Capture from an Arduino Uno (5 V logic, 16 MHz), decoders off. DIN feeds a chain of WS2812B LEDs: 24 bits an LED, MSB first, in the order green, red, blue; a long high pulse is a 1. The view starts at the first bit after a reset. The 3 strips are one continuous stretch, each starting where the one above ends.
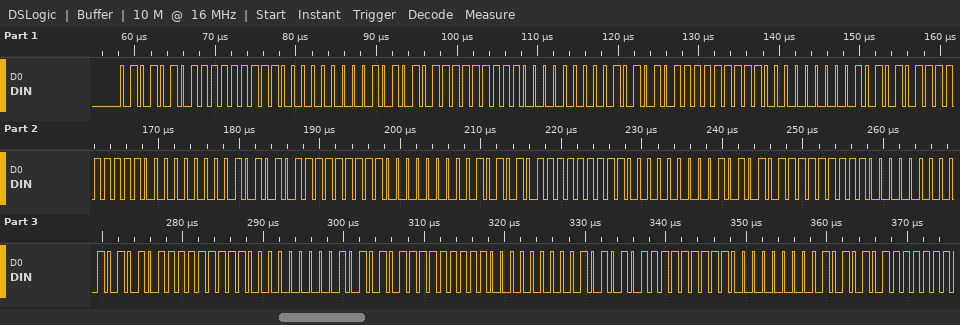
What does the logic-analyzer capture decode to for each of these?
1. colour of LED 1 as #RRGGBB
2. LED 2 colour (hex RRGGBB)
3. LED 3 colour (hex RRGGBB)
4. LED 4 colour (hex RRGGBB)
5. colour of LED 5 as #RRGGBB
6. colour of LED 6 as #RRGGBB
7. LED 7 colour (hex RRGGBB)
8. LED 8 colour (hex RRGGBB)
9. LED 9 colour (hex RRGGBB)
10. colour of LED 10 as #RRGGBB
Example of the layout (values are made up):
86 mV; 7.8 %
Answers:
#FF5500; #FF5500; #FF5500; #FF5500; #FF5500; #FF5500; #FF5500; #FF5500; #FF5500; #FF5500
